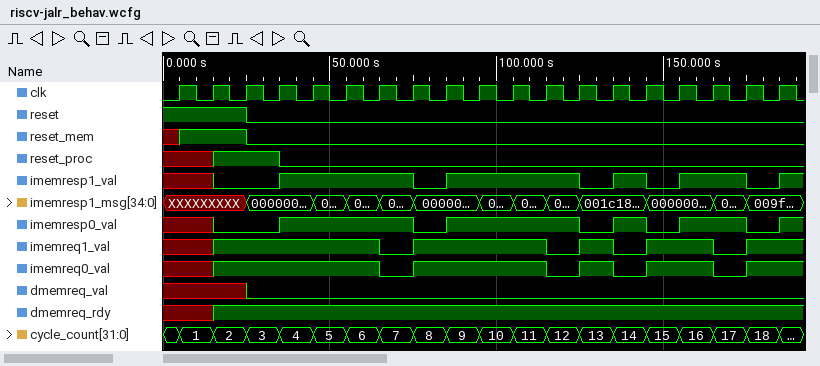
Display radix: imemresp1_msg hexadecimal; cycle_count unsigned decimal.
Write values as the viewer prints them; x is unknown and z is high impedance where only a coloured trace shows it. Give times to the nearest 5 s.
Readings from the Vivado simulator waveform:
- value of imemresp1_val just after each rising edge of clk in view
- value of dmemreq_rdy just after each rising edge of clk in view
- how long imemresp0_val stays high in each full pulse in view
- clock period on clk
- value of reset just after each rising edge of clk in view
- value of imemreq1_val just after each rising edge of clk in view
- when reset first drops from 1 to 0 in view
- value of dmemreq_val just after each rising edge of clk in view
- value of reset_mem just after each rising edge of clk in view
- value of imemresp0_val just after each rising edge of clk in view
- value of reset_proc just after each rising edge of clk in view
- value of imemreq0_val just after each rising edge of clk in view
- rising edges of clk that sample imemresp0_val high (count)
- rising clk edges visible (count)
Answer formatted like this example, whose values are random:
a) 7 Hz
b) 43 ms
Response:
a) x 0 0 1 1 1 1 0 1 1 1 1 0 1 0 1 1 0 1
b) x 1 1 1 1 1 1 1 1 1 1 1 1 1 1 1 1 1 1
c) 40 s, 40 s, 10 s, 20 s
d) 10 s
e) 1 1 0 0 0 0 0 0 0 0 0 0 0 0 0 0 0 0 0
f) x 1 1 1 1 1 0 1 1 1 1 0 1 0 1 1 0 1 1
g) 25 s
h) x x 0 0 0 0 0 0 0 0 0 0 0 0 0 0 0 0 0
i) 1 1 0 0 0 0 0 0 0 0 0 0 0 0 0 0 0 0 0
j) x 0 0 1 1 1 1 0 1 1 1 1 0 1 0 1 1 0 1
k) x 1 1 0 0 0 0 0 0 0 0 0 0 0 0 0 0 0 0
l) x 1 1 1 1 1 0 1 1 1 1 0 1 0 1 1 0 1 1
m) 11
n) 19
